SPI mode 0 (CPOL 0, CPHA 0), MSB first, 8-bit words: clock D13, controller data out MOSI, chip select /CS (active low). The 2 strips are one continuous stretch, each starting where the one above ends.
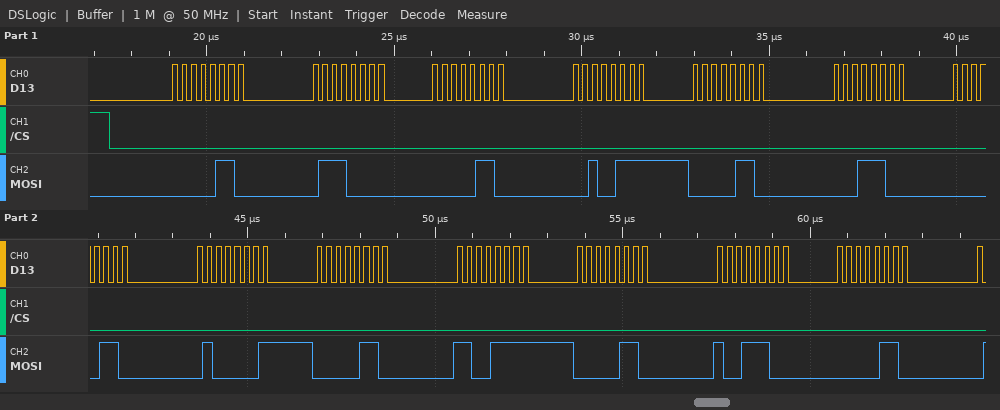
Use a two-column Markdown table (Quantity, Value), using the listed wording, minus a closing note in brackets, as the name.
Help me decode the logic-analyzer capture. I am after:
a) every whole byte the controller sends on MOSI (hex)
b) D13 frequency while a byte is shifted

| Quantity | Value |
|---|---|
| every whole byte the controller sends on MOSI | 0x06 0x70 0x06 0x27 0x06 0x1C 0x06 0x41 0x06 0xCF 0x06 0x9C 0x06 |
| D13 frequency while a byte is shifted | 4 MHz |
